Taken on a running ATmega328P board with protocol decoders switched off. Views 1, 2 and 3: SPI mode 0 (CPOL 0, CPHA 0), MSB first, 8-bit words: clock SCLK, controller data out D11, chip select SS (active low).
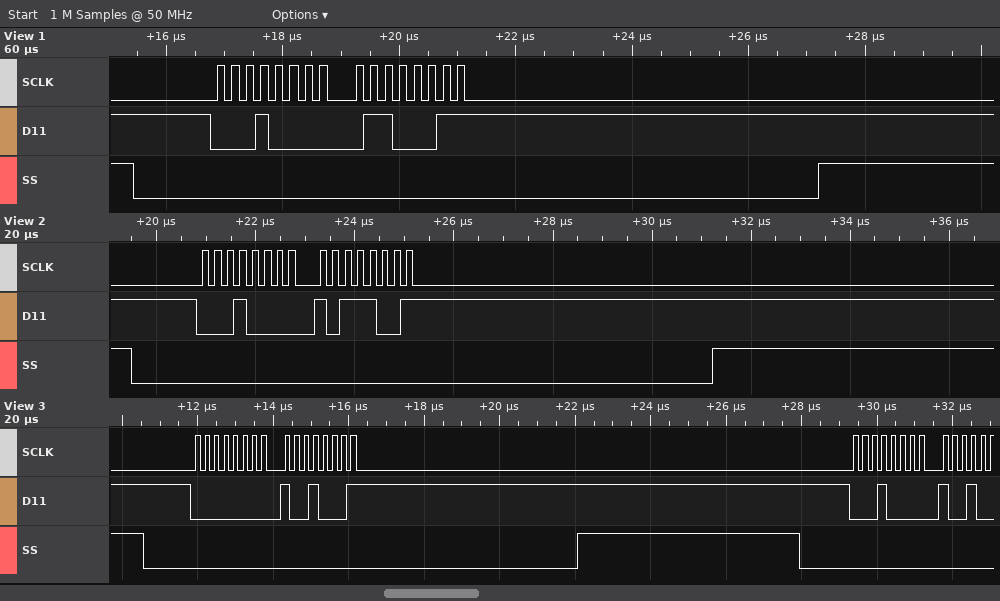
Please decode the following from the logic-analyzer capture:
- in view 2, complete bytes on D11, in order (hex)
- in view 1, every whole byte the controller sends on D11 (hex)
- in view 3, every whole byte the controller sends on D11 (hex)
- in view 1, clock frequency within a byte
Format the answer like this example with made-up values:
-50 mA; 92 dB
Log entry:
0x10 0xB9; 10 63; 00 91 10; 4 MHz
